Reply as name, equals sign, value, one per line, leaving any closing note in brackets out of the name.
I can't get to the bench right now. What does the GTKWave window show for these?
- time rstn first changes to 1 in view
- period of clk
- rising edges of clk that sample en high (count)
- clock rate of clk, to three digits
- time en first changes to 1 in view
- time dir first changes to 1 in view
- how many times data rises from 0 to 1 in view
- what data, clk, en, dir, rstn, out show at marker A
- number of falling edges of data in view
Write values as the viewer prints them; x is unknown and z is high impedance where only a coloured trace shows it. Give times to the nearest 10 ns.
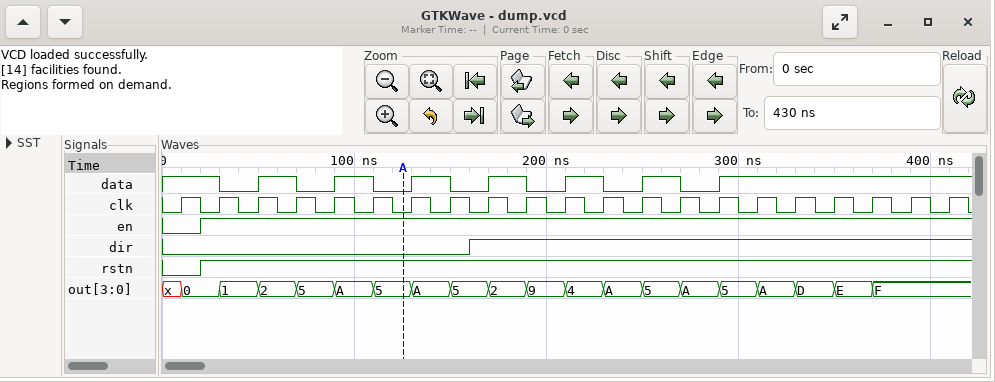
time rstn first changes to 1 in view = 20 ns
period of clk = 20 ns
rising edges of clk that sample en high = 20
clock rate of clk, to three digits = 50.0 MHz
time en first changes to 1 in view = 20 ns
time dir first changes to 1 in view = 160 ns
how many times data rises from 0 to 1 in view = 7
what data, clk, en, dir, rstn, out show at marker A = data=0, clk=0, en=1, dir=0, rstn=1, out=5
number of falling edges of data in view = 7
